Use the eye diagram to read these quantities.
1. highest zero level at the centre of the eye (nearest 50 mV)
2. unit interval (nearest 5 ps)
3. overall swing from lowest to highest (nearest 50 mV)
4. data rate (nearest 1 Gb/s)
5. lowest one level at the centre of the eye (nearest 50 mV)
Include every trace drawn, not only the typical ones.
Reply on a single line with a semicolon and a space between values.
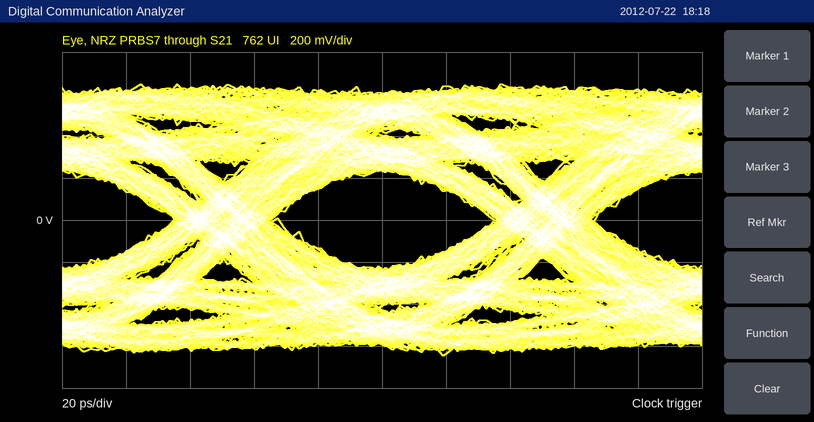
-250 mV; 100 ps; 1.30 V; 10 Gb/s; 250 mV
